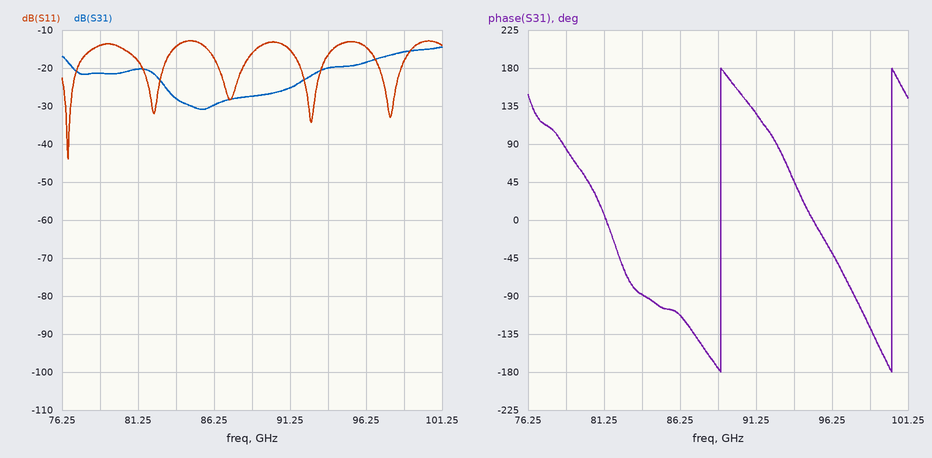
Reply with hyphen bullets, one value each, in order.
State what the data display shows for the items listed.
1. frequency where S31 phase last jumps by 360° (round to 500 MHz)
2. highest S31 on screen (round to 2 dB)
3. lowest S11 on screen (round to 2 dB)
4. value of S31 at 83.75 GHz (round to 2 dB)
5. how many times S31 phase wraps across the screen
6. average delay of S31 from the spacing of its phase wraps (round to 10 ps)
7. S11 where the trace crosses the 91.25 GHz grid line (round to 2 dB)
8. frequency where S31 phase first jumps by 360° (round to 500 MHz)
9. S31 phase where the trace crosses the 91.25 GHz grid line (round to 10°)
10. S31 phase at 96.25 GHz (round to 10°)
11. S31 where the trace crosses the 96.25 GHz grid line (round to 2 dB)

- 100.0 GHz
- -14 dB
- -44 dB
- -28 dB
- 2
- 90 ps
- -16 dB
- 89.0 GHz
- 130°
- -40°
- -18 dB
